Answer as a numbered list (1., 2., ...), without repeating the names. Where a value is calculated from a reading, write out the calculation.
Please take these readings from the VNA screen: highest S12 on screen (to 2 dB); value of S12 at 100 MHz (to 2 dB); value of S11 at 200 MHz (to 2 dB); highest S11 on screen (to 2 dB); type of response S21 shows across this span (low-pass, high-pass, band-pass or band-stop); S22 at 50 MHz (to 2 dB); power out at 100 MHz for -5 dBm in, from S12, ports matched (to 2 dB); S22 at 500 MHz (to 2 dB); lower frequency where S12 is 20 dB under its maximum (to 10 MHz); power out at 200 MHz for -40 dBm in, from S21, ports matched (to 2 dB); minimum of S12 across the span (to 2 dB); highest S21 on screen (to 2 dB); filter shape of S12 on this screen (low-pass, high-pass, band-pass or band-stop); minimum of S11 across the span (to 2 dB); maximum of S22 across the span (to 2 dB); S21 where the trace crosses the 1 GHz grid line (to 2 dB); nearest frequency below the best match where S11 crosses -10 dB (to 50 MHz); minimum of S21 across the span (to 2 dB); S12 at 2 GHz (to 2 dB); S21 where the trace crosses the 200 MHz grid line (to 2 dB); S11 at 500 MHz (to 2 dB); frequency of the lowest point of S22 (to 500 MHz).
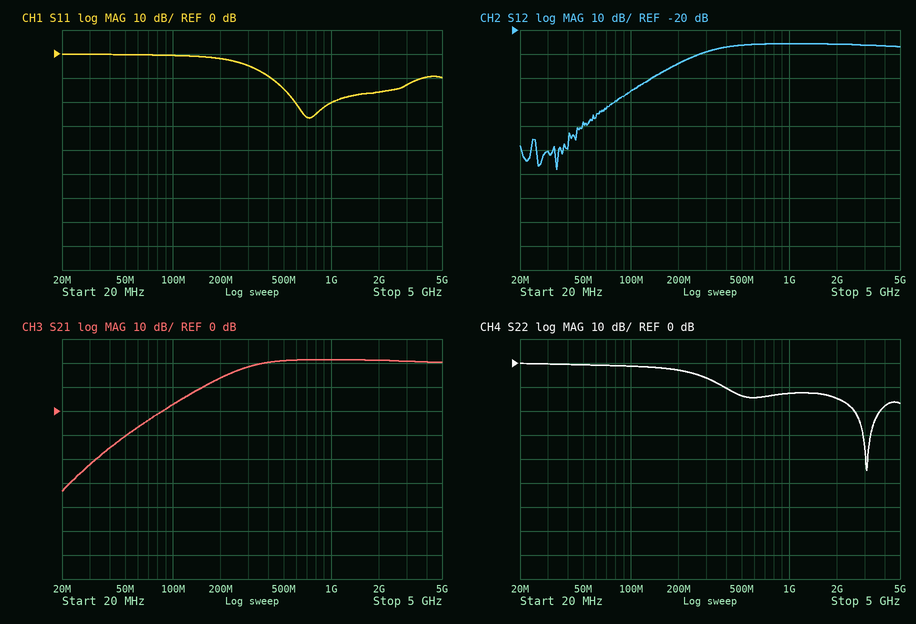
1. -26 dB
2. -46 dB
3. -2 dB
4. 0 dB
5. high-pass
6. 0 dB
7. -5 dBm + (-46 dB) = -50 dBm
8. -14 dB
9. 100 MHz
10. -40 dBm + (14 dB) = -26 dBm
11. -78 dB
12. 22 dB
13. high-pass
14. -26 dB
15. 0 dB
16. 22 dB
17. 400 MHz
18. -34 dB
19. -26 dB
20. 14 dB
21. -14 dB
22. 3.0 GHz
